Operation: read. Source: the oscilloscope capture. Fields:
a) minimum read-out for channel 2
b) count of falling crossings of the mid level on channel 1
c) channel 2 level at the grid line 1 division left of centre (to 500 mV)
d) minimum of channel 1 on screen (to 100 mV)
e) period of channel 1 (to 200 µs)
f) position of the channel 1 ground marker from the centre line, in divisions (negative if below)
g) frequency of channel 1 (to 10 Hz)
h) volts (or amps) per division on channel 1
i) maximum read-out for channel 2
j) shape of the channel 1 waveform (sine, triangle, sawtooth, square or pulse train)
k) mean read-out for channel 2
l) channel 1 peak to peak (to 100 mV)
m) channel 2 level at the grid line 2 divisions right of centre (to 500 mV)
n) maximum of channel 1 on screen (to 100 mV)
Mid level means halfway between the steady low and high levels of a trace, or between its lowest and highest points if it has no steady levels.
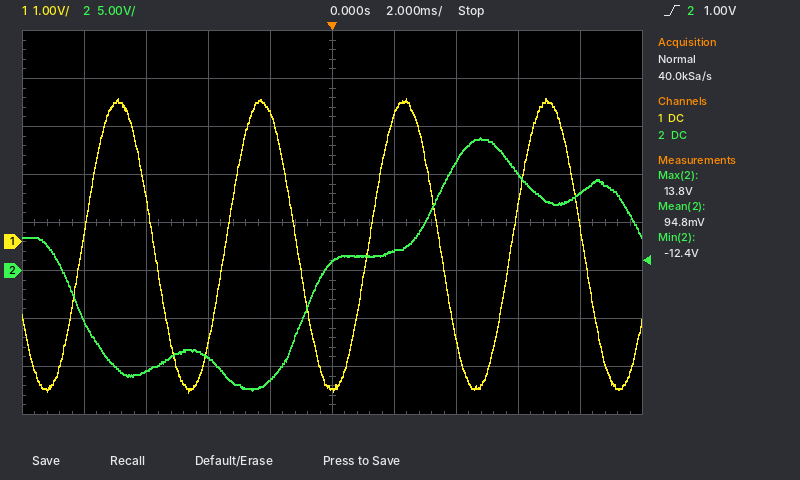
-12.4 V
4
-11.5 V
-3.1 V
4.6 ms
-0.4 div
220 Hz
1 V
13.8 V
sine
94.8 mV
6.1 V
11.5 V
3.0 V
